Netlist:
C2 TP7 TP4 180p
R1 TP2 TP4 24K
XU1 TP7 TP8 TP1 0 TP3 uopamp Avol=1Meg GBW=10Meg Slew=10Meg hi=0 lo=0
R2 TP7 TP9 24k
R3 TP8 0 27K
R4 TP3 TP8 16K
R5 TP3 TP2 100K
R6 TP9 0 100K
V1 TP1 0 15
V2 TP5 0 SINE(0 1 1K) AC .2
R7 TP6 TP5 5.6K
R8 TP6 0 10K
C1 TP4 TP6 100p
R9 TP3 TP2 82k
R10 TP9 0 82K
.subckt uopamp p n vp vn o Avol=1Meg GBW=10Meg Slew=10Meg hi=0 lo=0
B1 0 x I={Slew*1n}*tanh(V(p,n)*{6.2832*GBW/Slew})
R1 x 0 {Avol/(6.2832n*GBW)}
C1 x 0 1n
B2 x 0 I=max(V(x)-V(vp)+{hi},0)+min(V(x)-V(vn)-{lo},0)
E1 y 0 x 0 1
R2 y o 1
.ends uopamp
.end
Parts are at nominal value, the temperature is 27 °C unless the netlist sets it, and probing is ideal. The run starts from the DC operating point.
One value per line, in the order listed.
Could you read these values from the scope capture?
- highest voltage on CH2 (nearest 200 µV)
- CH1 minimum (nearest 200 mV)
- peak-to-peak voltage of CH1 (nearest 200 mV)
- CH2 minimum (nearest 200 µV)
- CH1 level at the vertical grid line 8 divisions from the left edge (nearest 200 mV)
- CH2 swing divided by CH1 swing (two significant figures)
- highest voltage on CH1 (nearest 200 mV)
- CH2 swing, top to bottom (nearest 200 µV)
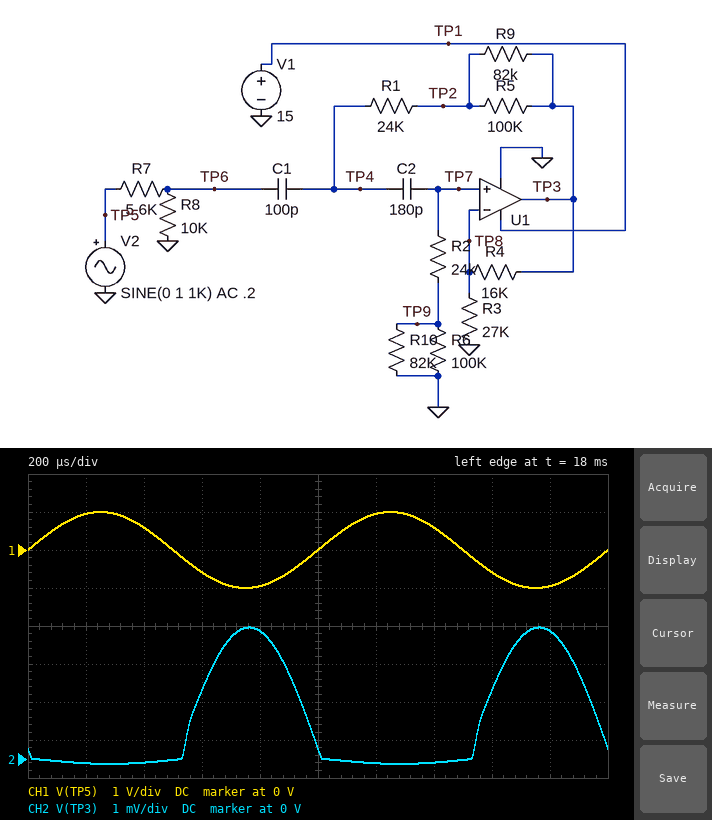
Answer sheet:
3.4 mV
-1.0 V
2.0 V
-200 µV
-600 mV
0.0018
1.0 V
3.6 mV
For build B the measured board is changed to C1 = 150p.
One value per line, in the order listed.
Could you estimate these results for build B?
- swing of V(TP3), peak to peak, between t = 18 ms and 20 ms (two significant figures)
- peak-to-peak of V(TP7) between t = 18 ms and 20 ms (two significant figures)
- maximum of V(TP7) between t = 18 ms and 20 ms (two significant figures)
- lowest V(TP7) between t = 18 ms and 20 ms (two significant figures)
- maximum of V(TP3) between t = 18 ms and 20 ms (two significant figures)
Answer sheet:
5.4 mV
6.5 mV
3.3 mV
-3.2 mV
5.2 mV
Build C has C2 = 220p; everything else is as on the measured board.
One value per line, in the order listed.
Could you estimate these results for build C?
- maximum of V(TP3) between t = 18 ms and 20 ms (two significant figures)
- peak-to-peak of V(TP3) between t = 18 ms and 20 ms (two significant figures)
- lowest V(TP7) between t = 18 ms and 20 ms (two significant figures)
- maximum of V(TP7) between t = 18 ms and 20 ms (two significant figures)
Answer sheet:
4.2 mV
4.4 mV
-2.6 mV
2.7 mV
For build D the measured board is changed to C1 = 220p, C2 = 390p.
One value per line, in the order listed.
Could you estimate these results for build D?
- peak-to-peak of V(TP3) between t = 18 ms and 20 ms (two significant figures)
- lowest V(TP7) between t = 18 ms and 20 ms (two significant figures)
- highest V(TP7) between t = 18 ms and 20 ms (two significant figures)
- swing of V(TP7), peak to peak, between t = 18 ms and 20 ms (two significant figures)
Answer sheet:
17 mV
-9.7 mV
10 mV
20 mV
